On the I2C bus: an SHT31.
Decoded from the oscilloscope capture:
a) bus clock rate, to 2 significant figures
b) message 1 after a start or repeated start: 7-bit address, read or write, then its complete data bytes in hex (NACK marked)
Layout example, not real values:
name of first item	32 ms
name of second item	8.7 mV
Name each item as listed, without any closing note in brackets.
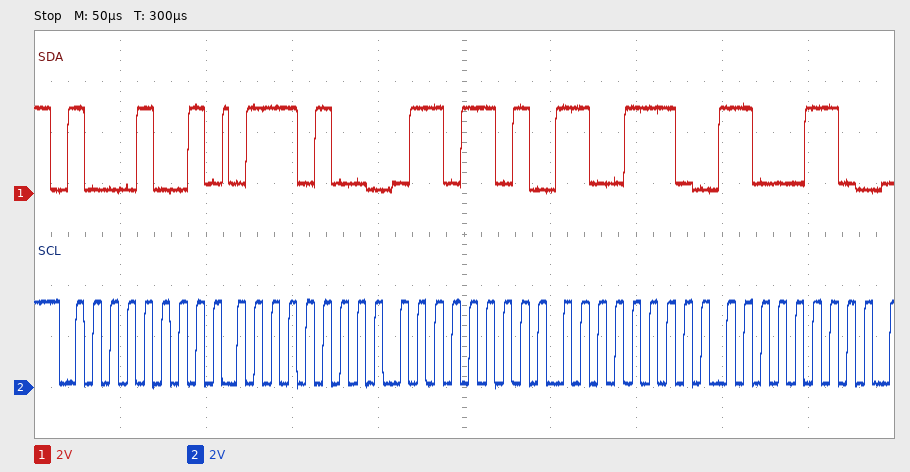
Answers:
bus clock rate, to 2 significant figures	100 kHz
message 1 after a start or repeated start: 7-bit address, read or write, then its complete data bytes in hex	0x44 read: 74 6D CE C6
